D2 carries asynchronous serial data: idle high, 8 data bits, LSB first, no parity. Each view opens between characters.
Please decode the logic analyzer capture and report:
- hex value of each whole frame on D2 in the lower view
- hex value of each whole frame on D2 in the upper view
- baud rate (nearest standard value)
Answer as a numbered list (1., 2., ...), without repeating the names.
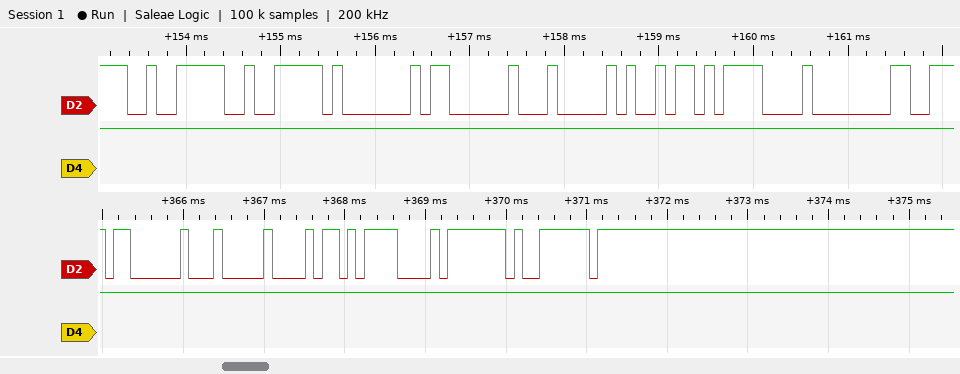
1. 03, 04, 68, 0F, 7F, 7E
2. F2, F2, 01, 03, 04, 69, 0F, 80
3. 9600 baud
